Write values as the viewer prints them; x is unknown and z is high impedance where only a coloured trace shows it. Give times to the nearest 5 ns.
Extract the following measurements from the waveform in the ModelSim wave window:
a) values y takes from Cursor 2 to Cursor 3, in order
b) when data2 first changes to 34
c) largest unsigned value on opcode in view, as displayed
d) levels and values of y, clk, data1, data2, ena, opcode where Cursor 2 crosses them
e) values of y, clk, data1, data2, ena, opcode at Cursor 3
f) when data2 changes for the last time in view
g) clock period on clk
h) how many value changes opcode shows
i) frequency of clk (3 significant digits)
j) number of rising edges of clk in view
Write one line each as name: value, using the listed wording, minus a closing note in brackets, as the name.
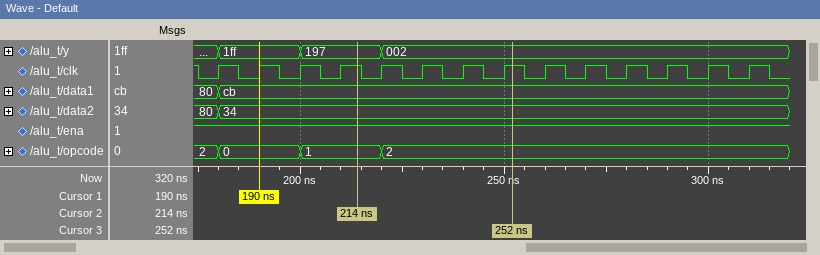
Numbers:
values y takes from Cursor 2 to Cursor 3, in order: 197, 002
when data2 first changes to 34: 180 ns
largest unsigned value on opcode in view, as displayed: 2
levels and values of y, clk, data1, data2, ena, opcode where Cursor 2 crosses them: y=197, clk=1, data1=cb, data2=34, ena=1, opcode=1
values of y, clk, data1, data2, ena, opcode at Cursor 3: y=002, clk=1, data1=cb, data2=34, ena=1, opcode=2
when data2 changes for the last time in view: 180 ns
clock period on clk: 10 ns
how many value changes opcode shows: 3
frequency of clk: 100 MHz
number of rising edges of clk in view: 14
